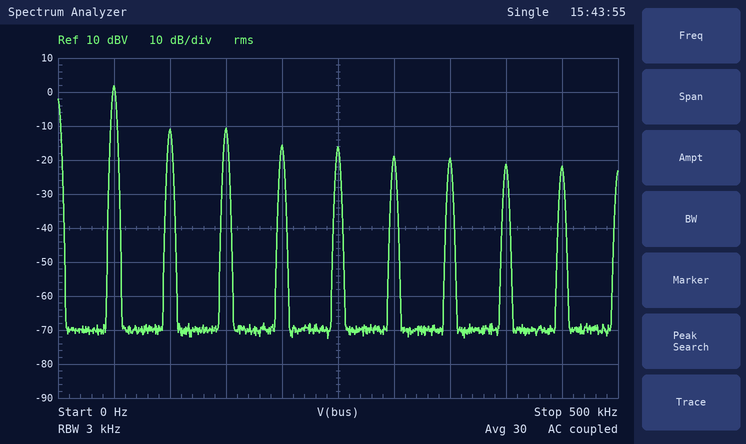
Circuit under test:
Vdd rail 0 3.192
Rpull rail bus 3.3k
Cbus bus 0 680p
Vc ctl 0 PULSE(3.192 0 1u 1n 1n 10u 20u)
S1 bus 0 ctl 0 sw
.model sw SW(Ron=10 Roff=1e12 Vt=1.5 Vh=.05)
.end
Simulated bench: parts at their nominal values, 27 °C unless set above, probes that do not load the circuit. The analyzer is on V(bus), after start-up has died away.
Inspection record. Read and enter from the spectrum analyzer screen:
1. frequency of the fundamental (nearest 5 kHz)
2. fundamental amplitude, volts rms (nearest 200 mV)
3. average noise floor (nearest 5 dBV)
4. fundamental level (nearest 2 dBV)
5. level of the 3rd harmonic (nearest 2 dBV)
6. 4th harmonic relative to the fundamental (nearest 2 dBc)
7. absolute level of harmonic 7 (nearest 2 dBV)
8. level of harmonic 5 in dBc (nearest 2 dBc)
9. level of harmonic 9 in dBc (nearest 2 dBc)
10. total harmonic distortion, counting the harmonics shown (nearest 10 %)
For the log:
50 kHz
1.2 V
-70 dBV
2 dBV
-10 dBV
-18 dBc
-20 dBV
-18 dBc
-24 dBc
40 %
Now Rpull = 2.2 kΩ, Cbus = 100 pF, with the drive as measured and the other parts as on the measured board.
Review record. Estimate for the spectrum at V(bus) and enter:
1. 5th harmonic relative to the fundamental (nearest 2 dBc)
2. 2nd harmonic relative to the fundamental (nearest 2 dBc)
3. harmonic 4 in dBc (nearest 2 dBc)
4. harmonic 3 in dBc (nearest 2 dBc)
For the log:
-14 dBc
-30 dBc
-30 dBc
-10 dBc
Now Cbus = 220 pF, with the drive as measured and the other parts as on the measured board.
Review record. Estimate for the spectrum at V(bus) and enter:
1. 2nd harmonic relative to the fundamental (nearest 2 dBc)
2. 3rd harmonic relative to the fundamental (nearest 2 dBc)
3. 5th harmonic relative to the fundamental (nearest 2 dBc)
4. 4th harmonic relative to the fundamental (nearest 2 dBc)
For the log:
-20 dBc
-10 dBc
-16 dBc
-22 dBc
